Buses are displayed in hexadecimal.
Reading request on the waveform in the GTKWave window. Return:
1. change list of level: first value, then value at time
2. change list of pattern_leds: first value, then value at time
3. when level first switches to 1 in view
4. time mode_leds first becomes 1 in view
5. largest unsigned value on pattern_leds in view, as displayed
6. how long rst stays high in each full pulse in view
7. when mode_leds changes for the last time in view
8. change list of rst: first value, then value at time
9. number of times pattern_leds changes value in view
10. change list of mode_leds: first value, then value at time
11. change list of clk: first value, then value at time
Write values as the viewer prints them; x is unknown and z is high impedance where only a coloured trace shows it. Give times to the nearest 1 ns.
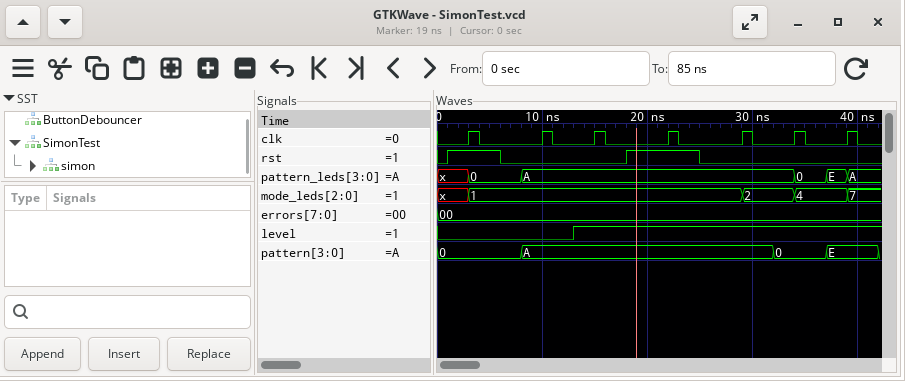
0, 1 at 13 ns
x, 0 at 3 ns, A at 8 ns, 0 at 34 ns, E at 37 ns, A at 39 ns
13 ns
3 ns
E
5 ns, 7 ns
39 ns
0, 1 at 1 ns, 0 at 6 ns, 1 at 18 ns, 0 at 25 ns
5
x, 1 at 3 ns, 2 at 29 ns, 4 at 34 ns, 7 at 39 ns
0, 1 at 3 ns, 0 at 4 ns, 1 at 10 ns, 0 at 11 ns, 1 at 15 ns, 0 at 16 ns, 1 at 22 ns, 0 at 23 ns, 1 at 29 ns, 0 at 30 ns, 1 at 34 ns, 0 at 35 ns, 1 at 39 ns, 0 at 40 ns
